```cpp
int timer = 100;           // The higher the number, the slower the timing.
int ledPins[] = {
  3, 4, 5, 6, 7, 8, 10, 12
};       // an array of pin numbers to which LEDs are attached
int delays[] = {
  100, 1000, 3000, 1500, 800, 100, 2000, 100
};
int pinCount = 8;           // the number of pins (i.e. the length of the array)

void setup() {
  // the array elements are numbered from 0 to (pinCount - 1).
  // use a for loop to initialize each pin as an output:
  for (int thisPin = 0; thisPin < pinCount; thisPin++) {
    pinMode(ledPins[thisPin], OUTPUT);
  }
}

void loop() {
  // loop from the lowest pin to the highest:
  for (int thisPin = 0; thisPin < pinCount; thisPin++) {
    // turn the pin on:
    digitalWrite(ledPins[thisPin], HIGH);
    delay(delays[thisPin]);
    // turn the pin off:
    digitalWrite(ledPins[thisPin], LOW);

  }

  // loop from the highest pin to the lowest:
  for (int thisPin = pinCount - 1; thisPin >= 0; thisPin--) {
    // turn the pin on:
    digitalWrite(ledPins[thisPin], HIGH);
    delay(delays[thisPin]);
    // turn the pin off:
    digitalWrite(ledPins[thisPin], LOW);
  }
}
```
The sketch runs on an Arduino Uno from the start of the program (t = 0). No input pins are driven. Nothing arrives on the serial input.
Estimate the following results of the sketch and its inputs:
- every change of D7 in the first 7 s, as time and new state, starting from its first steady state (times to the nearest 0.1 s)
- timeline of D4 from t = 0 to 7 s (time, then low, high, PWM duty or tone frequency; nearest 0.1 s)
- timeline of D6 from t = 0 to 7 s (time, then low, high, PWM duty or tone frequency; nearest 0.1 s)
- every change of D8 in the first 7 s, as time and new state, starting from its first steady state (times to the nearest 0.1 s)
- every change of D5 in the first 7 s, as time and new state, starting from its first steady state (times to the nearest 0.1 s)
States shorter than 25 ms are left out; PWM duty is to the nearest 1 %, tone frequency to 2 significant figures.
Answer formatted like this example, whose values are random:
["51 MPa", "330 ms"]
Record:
["0 s low; 5.6 s high; 6.4 s low", "0 s low; 0.1 s high; 1.1 s low", "0 s low; 4.1 s high; 5.6 s low", "0 s low; 6.4 s high; 6.5 s low", "0 s low; 1.1 s high; 4.1 s low"]
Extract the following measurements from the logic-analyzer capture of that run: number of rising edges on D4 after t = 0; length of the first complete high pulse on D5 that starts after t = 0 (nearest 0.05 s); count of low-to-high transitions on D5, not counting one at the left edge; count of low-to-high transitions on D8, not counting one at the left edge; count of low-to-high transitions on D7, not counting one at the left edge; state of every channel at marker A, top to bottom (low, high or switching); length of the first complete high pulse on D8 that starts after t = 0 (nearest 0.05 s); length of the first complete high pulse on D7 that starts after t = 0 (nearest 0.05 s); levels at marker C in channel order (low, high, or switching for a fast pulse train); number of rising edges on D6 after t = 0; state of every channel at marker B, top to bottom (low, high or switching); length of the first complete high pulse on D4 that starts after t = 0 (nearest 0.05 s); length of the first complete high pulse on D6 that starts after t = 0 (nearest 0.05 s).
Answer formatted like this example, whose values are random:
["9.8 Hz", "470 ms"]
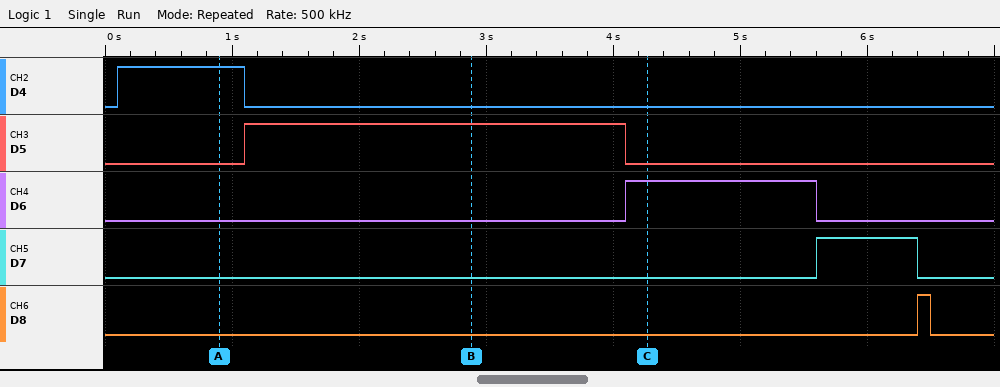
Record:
["1", "3.00 s", "1", "1", "1", "D4 high, D5 low, D6 low, D7 low, D8 low", "0.10 s", "0.80 s", "D4 low, D5 low, D6 high, D7 low, D8 low", "1", "D4 low, D5 high, D6 low, D7 low, D8 low", "1.00 s", "1.50 s"]
